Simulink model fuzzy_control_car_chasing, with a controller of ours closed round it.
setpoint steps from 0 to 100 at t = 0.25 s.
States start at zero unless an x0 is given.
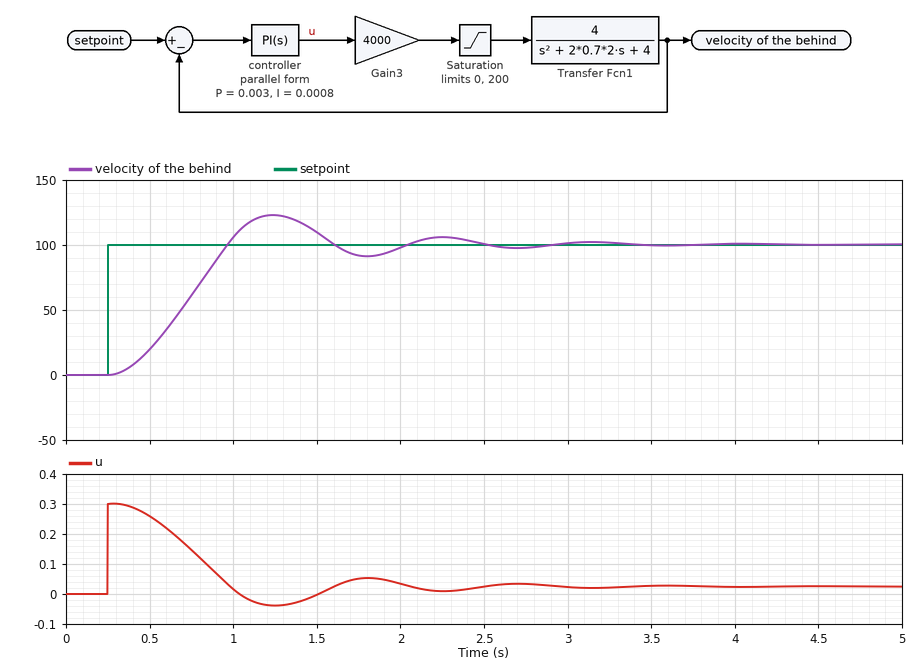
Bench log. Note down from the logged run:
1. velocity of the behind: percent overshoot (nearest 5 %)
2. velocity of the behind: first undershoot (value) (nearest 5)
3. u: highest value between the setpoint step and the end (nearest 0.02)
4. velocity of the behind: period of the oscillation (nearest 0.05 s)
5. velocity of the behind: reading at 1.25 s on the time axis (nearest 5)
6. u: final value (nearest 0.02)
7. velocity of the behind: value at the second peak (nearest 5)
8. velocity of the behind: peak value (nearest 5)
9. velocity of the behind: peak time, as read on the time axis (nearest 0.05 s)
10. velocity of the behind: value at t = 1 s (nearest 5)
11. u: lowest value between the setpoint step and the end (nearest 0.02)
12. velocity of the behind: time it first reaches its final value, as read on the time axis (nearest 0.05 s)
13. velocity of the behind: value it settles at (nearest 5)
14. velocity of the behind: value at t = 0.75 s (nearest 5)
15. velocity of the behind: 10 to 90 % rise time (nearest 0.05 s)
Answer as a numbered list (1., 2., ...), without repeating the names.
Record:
1. 25 %
2. 90
3. 0.30
4. 1.00 s
5. 125
6. 0.02
7. 105
8. 125
9. 1.25 s
10. 105
11. -0.04
12. 0.95 s
13. 100
14. 60
15. 0.50 s
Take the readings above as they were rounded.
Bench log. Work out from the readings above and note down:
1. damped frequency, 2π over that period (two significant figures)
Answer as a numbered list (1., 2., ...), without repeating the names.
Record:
1. 6.3 rad/s
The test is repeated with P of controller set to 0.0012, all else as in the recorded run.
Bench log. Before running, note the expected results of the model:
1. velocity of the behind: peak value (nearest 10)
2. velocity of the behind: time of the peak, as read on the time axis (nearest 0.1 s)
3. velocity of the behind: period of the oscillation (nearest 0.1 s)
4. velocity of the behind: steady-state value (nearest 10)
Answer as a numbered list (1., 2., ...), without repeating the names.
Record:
1. 130
2. 1.3 s
3. 1.4 s
4. 100
